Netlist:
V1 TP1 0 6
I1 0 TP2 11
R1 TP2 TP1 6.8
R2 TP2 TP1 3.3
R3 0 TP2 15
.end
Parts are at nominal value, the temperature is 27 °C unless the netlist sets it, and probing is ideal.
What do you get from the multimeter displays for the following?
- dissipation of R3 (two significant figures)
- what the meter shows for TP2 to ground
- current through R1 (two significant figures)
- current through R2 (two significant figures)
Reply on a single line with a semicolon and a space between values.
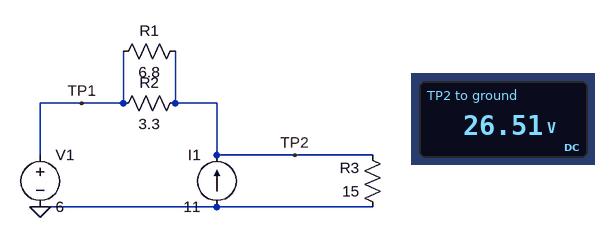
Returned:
47 W; 26.51 V; 3.0 A; 6.2 A
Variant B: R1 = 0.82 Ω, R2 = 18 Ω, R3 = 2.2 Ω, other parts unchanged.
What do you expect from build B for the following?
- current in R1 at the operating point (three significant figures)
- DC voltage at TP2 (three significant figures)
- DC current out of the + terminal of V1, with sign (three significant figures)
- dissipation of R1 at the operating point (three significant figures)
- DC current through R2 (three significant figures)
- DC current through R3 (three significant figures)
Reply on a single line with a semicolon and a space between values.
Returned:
5.83 A; 10.8 V; -6.10 A; 27.9 W; 266 mA; 4.90 A
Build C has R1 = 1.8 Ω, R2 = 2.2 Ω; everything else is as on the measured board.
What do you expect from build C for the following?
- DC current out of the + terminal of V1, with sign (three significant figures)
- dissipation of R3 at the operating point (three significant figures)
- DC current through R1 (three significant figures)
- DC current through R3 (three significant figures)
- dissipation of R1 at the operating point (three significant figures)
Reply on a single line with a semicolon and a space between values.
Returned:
-9.94 A; 16.7 W; 5.47 A; 1.06 A; 53.8 W
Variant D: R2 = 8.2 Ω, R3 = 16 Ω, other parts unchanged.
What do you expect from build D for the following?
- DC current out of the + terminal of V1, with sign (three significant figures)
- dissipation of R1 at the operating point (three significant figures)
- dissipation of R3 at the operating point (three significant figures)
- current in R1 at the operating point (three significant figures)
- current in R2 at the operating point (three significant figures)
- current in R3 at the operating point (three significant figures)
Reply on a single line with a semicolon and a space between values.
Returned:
-8.62 A; 151 W; 90.5 W; 4.71 A; 3.91 A; 2.38 A
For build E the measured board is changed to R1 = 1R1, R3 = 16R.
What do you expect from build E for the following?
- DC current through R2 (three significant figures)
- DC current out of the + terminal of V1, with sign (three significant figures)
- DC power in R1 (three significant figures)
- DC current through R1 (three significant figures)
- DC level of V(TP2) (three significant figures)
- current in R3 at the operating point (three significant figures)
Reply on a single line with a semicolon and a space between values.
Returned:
2.53 A; -10.1 A; 63.2 W; 7.58 A; 14.3 V; 896 mA
